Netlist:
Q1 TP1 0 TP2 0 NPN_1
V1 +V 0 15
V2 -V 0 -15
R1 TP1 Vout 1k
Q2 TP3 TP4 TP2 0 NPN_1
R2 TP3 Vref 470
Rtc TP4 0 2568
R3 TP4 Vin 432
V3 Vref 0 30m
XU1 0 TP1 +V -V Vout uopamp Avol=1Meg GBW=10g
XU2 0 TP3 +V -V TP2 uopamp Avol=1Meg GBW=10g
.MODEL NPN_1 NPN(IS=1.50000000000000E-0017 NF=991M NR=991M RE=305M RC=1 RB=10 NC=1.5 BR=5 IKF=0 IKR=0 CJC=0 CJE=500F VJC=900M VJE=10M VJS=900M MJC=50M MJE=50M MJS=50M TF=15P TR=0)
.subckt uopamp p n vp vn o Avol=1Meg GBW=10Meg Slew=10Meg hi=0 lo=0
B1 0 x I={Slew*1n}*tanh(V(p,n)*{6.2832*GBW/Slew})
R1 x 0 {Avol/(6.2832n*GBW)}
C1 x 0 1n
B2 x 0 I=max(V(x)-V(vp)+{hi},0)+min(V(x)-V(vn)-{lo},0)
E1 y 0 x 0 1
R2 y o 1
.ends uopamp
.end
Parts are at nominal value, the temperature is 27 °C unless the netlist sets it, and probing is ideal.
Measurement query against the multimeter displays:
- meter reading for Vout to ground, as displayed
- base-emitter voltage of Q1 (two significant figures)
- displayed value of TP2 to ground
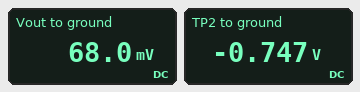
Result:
68.0 mV
750 mV
-0.747 V
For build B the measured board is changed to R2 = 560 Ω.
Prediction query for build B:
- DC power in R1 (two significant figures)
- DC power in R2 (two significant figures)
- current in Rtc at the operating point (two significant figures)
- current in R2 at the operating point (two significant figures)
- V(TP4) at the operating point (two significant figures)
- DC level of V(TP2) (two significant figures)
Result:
3.2 µW
1.6 µW
540 nA
54 µA
-1.4 mV
-740 mV
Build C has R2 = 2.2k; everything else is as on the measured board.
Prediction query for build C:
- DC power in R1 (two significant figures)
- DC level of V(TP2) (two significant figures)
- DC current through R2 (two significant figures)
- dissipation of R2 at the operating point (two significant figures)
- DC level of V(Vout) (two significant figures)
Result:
190 nW
-710 mV
14 µA
410 nW
14 mV
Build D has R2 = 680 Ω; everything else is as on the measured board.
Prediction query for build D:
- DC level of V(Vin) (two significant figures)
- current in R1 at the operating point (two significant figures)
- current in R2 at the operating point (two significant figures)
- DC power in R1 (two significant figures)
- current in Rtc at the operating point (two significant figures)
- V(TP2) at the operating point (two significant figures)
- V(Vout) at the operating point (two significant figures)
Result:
-1.1 mV
46 µA
44 µA
2.1 µW
440 nA
-740 mV
46 mV
